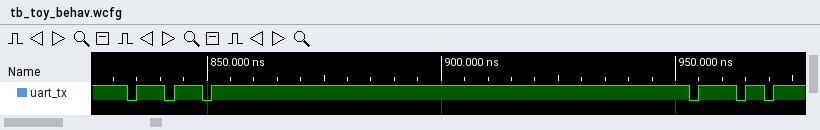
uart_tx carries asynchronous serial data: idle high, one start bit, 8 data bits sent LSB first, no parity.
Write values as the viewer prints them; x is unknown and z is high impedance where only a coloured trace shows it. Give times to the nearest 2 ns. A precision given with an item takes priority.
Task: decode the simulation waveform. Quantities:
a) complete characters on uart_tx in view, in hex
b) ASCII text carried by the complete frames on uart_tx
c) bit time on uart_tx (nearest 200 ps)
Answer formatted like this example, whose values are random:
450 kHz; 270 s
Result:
77, 6F; "wo"; 2000 ps
